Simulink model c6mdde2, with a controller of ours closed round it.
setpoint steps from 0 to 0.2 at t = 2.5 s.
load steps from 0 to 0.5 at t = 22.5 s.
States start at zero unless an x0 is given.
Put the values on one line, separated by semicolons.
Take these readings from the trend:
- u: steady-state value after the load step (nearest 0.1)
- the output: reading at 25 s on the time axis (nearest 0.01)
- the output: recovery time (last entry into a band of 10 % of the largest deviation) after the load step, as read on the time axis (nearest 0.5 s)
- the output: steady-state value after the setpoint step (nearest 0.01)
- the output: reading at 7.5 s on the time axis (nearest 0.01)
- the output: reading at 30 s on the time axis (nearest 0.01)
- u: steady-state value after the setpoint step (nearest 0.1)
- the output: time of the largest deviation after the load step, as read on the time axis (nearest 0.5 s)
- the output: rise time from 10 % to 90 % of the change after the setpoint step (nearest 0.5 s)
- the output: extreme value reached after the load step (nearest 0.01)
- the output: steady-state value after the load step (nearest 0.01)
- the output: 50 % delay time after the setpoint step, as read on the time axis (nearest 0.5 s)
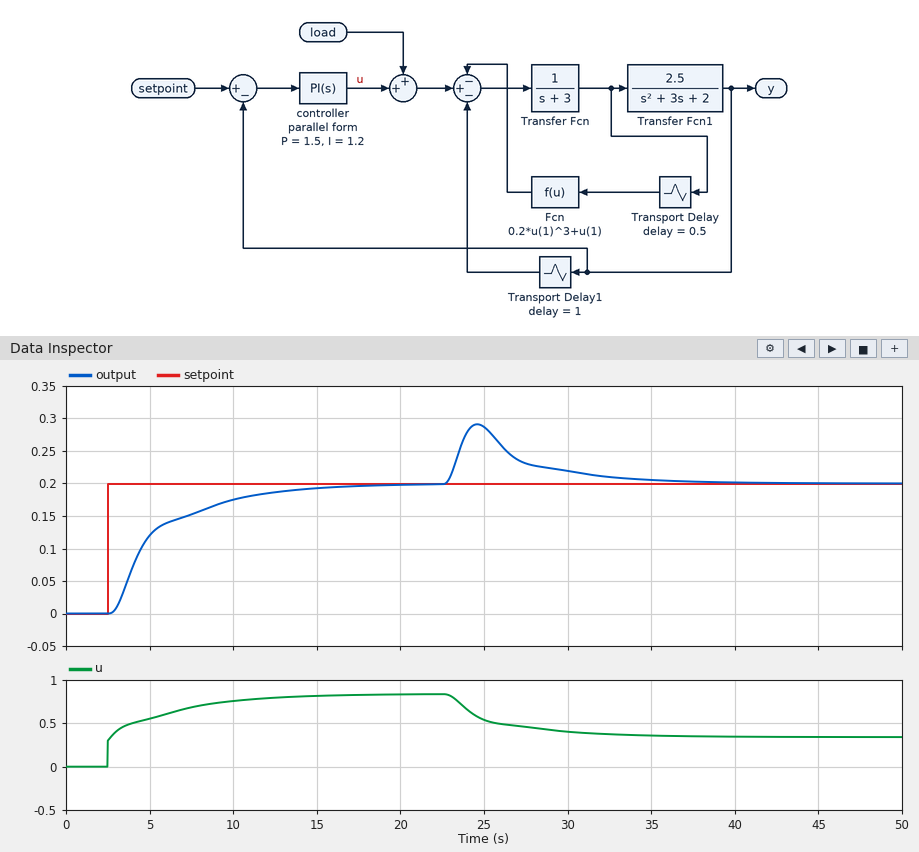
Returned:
0.3; 0.29; 33.0 s; 0.20; 0.15; 0.22; 0.8; 24.5 s; 7.5 s; 0.29; 0.20; 4.5 s
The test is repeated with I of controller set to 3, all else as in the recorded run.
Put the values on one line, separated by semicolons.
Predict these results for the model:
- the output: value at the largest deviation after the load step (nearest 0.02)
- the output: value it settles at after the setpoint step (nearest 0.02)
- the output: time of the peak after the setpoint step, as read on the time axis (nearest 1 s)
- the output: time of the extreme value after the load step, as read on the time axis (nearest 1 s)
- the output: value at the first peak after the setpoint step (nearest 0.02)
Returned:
0.28; 0.20; 6 s; 24 s; 0.22
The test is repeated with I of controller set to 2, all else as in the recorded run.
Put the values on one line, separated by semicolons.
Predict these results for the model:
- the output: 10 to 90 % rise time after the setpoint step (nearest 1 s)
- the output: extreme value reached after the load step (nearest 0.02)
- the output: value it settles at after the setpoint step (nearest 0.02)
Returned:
3 s; 0.28; 0.20
